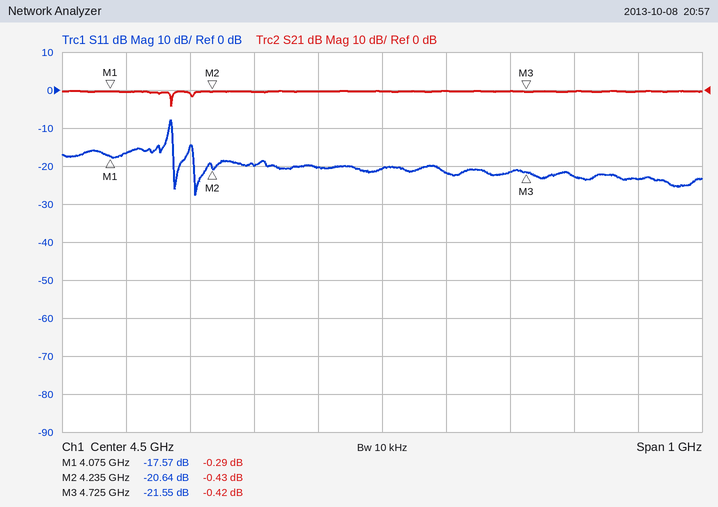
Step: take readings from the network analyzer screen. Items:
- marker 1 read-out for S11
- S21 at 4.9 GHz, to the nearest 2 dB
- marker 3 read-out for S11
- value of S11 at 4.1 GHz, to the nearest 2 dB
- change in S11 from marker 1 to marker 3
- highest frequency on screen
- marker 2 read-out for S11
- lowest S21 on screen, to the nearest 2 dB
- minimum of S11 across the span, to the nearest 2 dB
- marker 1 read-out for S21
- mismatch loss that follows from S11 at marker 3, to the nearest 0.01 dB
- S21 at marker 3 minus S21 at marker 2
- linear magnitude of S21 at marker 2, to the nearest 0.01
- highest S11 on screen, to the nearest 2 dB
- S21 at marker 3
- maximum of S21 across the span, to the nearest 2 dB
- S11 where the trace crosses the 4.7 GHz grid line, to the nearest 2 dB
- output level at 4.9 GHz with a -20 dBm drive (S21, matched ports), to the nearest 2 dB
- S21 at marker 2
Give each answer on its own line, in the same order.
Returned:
-17.57 dB
0 dB
-21.55 dB
-16 dB
-3.98 dB
5 GHz
-20.64 dB
-4 dB
-28 dB
-0.29 dB
0.03 dB
0.01 dB
0.95
-8 dB
-0.42 dB
0 dB
-22 dB
-20 dBm
-0.43 dB
